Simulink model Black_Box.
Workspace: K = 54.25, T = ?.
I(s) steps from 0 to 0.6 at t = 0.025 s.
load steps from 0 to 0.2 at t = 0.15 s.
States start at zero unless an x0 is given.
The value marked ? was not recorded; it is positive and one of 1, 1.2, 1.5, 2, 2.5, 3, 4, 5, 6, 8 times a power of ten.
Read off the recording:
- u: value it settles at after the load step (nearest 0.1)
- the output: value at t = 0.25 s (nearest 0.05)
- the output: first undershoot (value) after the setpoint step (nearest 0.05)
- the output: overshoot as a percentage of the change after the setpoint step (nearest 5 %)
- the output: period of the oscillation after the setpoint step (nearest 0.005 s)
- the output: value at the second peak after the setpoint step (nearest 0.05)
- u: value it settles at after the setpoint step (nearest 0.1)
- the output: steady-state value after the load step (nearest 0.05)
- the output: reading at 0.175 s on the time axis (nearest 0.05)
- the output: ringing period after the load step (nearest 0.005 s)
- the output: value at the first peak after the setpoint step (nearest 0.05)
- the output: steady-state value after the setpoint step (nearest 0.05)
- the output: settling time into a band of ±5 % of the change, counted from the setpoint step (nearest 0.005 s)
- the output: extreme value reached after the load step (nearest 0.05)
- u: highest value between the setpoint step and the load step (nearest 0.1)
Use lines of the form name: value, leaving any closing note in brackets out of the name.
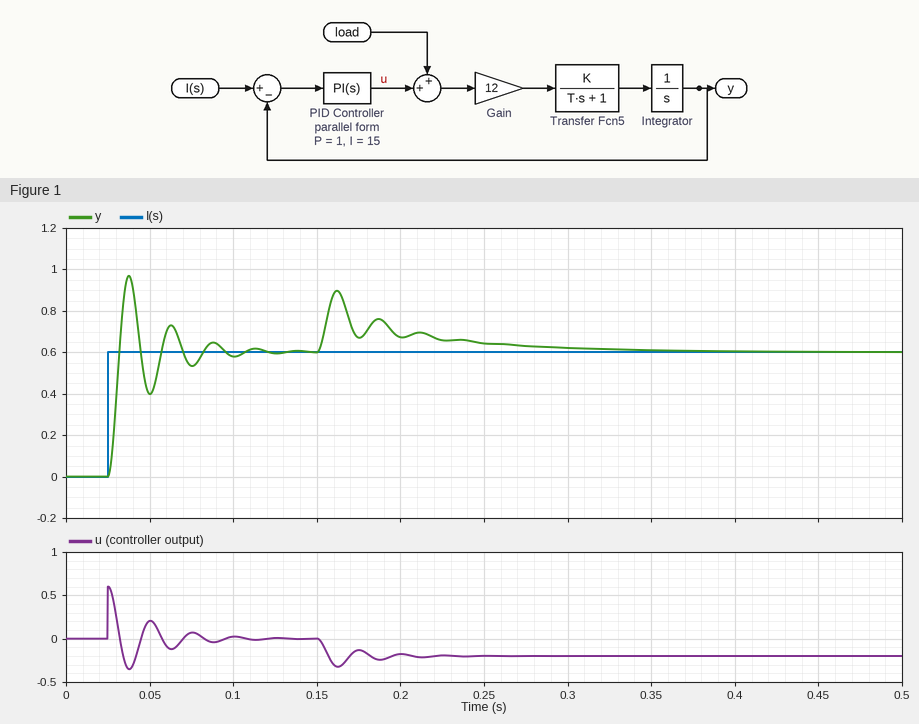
u: value it settles at after the load step: -0.2
the output: value at t = 0.25 s: 0.65
the output: first undershoot (value) after the setpoint step: 0.40
the output: overshoot as a percentage of the change after the setpoint step: 60 %
the output: period of the oscillation after the setpoint step: 0.025 s
the output: value at the second peak after the setpoint step: 0.75
u: value it settles at after the setpoint step: 0.0
the output: steady-state value after the load step: 0.60
the output: reading at 0.175 s on the time axis: 0.65
the output: ringing period after the load step: 0.025 s
the output: value at the first peak after the setpoint step: 0.95
the output: steady-state value after the setpoint step: 0.60
the output: settling time into a band of ±5 % of the change, counted from the setpoint step: 0.065 s
the output: extreme value reached after the load step: 0.90
u: highest value between the setpoint step and the load step: 0.6
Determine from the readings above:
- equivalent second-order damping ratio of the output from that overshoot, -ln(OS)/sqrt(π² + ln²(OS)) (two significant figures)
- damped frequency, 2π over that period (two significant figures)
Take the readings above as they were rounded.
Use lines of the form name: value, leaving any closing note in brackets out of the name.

equivalent second-order damping ratio of the output from that overshoot, -ln(OS)/sqrt(π² + ln²(OS)): 0.16
damped frequency, 2π over that period: 250 rad/s
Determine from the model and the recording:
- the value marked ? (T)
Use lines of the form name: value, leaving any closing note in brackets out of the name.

the value marked ?: 0.01
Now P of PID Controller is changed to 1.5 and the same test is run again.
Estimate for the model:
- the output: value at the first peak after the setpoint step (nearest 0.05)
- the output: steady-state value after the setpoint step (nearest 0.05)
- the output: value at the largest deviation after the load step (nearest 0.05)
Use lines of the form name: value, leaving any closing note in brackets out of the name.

the output: value at the first peak after the setpoint step: 1.00
the output: steady-state value after the setpoint step: 0.60
the output: value at the largest deviation after the load step: 0.80
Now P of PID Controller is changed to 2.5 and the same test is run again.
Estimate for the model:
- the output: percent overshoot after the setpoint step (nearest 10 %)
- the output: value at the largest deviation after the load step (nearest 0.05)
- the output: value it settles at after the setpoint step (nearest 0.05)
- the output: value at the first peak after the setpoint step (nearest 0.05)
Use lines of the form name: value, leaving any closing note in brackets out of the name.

the output: percent overshoot after the setpoint step: 70 %
the output: value at the largest deviation after the load step: 0.75
the output: value it settles at after the setpoint step: 0.60
the output: value at the first peak after the setpoint step: 1.00
